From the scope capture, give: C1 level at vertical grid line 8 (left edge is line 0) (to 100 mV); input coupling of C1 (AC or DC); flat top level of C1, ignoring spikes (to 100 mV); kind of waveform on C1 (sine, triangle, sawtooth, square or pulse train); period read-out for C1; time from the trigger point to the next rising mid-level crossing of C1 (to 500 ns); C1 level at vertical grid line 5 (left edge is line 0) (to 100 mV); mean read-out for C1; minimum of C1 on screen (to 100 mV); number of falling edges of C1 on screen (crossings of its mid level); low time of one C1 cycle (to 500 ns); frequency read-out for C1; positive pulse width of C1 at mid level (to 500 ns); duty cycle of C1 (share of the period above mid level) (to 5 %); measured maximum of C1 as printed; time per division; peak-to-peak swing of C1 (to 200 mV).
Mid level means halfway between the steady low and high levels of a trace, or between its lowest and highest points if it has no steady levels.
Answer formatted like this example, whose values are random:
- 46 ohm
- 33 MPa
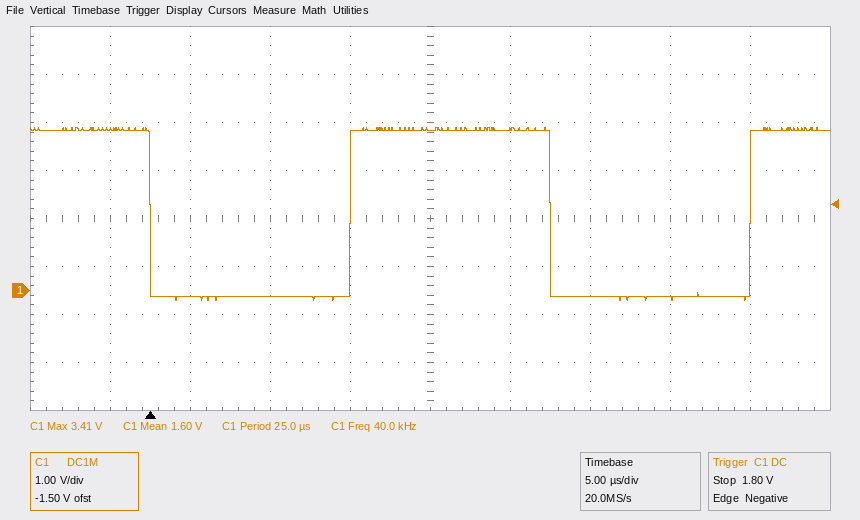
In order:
- -200 mV
- DC
- 3.3 V
- square
- 25.0 µs
- 12.5 µs
- 3.4 V
- 1.60 V
- -200 mV
- 2
- 12.5 µs
- 40.0 kHz
- 12.5 µs
- 50 %
- 3.41 V
- 5 µs
- 3.6 V
